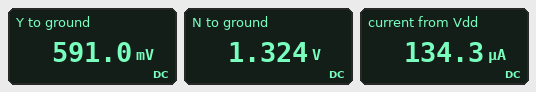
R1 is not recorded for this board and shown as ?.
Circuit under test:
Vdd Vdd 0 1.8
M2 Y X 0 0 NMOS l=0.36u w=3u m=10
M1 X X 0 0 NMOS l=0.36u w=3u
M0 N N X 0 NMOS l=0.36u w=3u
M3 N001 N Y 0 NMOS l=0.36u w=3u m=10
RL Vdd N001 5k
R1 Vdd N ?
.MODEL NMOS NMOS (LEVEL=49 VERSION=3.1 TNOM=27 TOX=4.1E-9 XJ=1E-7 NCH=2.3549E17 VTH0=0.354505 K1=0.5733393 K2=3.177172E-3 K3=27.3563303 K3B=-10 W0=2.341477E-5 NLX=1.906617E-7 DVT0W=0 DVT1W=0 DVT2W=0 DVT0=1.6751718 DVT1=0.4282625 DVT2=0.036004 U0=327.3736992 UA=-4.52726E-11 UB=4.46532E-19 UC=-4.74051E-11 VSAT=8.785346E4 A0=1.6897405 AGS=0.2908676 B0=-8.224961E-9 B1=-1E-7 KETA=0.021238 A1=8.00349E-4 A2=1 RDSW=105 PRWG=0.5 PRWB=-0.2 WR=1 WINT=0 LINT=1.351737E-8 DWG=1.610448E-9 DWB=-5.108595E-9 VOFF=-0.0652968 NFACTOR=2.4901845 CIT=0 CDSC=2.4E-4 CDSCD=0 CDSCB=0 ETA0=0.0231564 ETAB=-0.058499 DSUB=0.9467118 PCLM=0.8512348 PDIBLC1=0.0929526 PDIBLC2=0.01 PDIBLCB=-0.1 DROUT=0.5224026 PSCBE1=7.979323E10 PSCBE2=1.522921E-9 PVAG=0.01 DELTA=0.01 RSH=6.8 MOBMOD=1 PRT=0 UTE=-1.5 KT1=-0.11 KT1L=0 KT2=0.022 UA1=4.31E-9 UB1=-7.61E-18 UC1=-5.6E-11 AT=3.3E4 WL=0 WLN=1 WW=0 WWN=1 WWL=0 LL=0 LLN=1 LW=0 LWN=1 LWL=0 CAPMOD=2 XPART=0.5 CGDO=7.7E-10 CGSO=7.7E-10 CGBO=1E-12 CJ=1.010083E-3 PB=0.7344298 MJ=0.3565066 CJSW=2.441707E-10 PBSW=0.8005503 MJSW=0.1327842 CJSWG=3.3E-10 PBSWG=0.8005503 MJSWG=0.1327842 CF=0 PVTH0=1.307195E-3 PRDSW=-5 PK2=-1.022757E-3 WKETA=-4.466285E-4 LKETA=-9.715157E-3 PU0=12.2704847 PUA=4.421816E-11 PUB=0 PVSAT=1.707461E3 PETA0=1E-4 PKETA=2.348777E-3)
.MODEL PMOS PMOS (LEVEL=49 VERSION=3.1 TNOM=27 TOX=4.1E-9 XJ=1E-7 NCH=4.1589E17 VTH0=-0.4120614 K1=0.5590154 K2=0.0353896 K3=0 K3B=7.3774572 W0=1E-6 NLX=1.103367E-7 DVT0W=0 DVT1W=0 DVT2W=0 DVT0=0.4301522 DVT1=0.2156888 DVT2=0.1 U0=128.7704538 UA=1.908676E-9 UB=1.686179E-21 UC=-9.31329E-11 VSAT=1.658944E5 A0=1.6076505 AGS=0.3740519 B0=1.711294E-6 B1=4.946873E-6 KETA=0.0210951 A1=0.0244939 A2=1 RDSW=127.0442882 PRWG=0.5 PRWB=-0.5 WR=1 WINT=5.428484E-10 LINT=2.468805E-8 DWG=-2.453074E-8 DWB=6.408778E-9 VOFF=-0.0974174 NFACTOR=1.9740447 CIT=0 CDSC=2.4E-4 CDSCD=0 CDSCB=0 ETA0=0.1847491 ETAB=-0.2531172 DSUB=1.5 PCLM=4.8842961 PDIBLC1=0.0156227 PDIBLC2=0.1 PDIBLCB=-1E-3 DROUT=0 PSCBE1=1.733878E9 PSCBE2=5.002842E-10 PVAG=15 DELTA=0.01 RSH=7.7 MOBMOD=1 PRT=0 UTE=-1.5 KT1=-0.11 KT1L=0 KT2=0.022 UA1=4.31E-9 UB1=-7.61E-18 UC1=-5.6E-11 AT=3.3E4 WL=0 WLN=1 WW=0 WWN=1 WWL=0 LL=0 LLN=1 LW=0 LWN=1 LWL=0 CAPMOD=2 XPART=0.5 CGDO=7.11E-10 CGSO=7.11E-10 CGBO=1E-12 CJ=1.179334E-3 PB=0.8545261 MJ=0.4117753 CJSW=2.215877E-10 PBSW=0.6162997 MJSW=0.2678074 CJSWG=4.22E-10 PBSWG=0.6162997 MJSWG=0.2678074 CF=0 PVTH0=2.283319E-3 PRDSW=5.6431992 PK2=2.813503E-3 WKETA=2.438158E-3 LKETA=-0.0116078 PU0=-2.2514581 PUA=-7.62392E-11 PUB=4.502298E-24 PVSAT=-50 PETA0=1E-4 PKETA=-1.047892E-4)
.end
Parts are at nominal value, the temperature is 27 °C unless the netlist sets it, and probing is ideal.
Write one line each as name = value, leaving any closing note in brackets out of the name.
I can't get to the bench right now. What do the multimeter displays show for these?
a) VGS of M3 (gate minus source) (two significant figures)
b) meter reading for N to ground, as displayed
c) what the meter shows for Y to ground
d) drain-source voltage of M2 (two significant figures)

VGS of M3 (gate minus source) = 730 mV
meter reading for N to ground, as displayed = 1.324 V
what the meter shows for Y to ground = 591.0 mV
drain-source voltage of M2 = 590 mV
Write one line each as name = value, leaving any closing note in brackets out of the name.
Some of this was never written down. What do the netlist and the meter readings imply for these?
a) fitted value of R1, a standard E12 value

fitted value of R1, a standard E12 value = 39 kΩ
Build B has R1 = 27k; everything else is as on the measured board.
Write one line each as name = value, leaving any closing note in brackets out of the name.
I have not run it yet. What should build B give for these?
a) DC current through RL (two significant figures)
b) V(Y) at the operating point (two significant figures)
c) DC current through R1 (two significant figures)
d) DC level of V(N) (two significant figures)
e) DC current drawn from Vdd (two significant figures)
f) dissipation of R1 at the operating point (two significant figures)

DC current through RL = 160 µA
V(Y) at the operating point = 610 mV
DC current through R1 = 16 µA
DC level of V(N) = 1.4 V
DC current drawn from Vdd = 180 µA
dissipation of R1 at the operating point = 7.1 µW
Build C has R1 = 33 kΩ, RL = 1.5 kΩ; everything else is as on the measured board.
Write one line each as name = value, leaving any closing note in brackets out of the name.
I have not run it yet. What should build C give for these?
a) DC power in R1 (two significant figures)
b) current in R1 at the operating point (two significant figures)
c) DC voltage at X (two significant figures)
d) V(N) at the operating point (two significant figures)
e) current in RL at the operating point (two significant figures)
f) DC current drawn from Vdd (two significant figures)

DC power in R1 = 6.4 µW
current in R1 at the operating point = 14 µA
DC voltage at X = 600 mV
V(N) at the operating point = 1.3 V
current in RL at the operating point = 140 µA
DC current drawn from Vdd = 150 µA
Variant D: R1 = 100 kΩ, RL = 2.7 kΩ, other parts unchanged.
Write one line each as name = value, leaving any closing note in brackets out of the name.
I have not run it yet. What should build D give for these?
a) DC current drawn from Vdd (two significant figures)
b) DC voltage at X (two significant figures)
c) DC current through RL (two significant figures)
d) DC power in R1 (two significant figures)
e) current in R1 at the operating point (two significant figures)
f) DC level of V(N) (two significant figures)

DC current drawn from Vdd = 62 µA
DC voltage at X = 550 mV
DC current through RL = 57 µA
DC power in R1 = 3.2 µW
current in R1 at the operating point = 5.7 µA
DC level of V(N) = 1.2 V
